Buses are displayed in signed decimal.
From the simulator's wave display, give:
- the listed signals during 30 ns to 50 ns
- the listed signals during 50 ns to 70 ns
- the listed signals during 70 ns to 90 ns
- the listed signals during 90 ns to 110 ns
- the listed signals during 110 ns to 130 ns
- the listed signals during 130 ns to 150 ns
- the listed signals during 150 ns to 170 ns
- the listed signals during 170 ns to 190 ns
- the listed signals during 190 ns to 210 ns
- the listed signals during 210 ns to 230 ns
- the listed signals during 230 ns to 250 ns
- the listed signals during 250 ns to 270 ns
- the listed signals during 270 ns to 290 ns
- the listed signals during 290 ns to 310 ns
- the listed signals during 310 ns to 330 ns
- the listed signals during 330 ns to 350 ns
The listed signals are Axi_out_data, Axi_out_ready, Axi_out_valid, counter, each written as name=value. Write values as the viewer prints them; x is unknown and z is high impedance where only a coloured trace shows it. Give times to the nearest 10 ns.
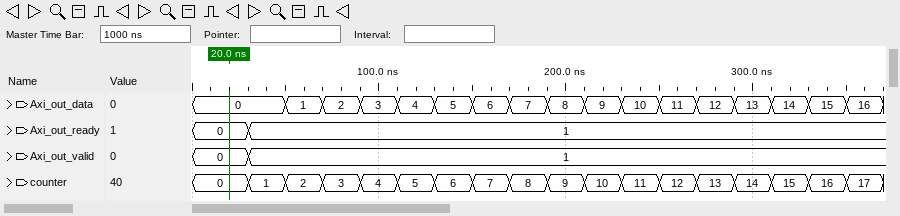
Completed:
Axi_out_data=0, Axi_out_ready=1, Axi_out_valid=1, counter=1
Axi_out_data=1, Axi_out_ready=1, Axi_out_valid=1, counter=2
Axi_out_data=2, Axi_out_ready=1, Axi_out_valid=1, counter=3
Axi_out_data=3, Axi_out_ready=1, Axi_out_valid=1, counter=4
Axi_out_data=4, Axi_out_ready=1, Axi_out_valid=1, counter=5
Axi_out_data=5, Axi_out_ready=1, Axi_out_valid=1, counter=6
Axi_out_data=6, Axi_out_ready=1, Axi_out_valid=1, counter=7
Axi_out_data=7, Axi_out_ready=1, Axi_out_valid=1, counter=8
Axi_out_data=8, Axi_out_ready=1, Axi_out_valid=1, counter=9
Axi_out_data=9, Axi_out_ready=1, Axi_out_valid=1, counter=10
Axi_out_data=10, Axi_out_ready=1, Axi_out_valid=1, counter=11
Axi_out_data=11, Axi_out_ready=1, Axi_out_valid=1, counter=12
Axi_out_data=12, Axi_out_ready=1, Axi_out_valid=1, counter=13
Axi_out_data=13, Axi_out_ready=1, Axi_out_valid=1, counter=14
Axi_out_data=14, Axi_out_ready=1, Axi_out_valid=1, counter=15
Axi_out_data=15, Axi_out_ready=1, Axi_out_valid=1, counter=16
